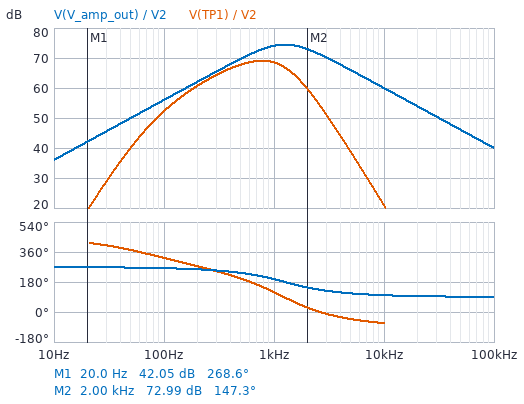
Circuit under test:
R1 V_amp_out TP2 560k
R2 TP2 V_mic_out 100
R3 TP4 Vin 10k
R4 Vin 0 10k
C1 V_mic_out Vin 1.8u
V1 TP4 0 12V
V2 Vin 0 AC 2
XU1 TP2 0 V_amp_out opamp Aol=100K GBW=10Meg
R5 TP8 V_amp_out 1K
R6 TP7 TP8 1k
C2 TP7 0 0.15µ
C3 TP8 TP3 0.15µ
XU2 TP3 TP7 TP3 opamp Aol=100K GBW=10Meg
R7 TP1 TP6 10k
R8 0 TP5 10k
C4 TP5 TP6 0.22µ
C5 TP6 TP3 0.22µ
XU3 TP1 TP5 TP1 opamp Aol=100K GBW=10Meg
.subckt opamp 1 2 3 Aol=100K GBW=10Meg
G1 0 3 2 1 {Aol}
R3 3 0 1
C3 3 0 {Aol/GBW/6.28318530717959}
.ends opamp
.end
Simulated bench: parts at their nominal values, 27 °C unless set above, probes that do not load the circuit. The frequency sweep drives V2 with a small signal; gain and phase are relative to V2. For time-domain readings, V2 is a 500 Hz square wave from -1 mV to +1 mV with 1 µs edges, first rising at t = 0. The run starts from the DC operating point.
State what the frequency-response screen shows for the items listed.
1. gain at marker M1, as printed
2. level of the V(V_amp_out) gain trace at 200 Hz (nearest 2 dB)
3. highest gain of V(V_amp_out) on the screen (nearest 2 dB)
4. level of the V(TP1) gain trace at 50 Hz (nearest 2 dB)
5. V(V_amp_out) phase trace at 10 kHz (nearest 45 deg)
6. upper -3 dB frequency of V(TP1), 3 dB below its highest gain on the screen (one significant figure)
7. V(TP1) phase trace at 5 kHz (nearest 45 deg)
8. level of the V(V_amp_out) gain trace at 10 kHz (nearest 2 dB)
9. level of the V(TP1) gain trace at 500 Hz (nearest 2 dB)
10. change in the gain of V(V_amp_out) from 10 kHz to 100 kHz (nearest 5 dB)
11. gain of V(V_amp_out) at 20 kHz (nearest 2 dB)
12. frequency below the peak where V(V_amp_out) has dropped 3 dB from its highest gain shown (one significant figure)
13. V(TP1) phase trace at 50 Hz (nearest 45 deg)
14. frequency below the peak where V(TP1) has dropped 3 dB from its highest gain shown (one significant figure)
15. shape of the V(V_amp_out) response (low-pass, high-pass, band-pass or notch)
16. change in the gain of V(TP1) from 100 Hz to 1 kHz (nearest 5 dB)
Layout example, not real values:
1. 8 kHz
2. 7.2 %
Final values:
1. 42.05 dB
2. 62 dB
3. 74 dB
4. 40 dB
5. 90 deg
6. 1 kHz
7. -45 deg
8. 60 dB
9. 68 dB
10. -20 dB
11. 54 dB
12. 600 Hz
13. 360 deg
14. 400 Hz
15. band-pass
16. 15 dB
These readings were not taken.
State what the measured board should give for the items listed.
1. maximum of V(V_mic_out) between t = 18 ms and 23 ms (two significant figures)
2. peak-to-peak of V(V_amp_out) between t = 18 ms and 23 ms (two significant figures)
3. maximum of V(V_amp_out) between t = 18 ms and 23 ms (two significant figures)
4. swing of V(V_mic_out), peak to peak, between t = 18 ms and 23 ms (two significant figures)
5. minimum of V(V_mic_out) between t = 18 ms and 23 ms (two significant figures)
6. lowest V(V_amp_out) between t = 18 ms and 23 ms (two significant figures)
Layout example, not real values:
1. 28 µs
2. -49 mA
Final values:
1. 2.0 mV
2. 14 V
3. 7.0 V
4. 4.0 mV
5. -2.0 mV
6. -7.0 V
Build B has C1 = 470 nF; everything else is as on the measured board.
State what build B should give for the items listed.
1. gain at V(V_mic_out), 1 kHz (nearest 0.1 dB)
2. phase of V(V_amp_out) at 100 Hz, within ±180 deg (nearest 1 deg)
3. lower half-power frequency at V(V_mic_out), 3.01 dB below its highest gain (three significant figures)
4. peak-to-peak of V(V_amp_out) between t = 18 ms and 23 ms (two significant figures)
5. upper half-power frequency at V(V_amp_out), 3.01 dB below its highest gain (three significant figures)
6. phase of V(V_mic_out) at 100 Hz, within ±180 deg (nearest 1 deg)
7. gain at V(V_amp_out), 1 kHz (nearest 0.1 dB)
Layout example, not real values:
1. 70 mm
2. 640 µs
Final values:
1. -8.0 dB
2. -92 deg
3. 1.92 kHz
4. 10 V
5. 3.58 kHz
6. 91 deg
7. 65.4 dB
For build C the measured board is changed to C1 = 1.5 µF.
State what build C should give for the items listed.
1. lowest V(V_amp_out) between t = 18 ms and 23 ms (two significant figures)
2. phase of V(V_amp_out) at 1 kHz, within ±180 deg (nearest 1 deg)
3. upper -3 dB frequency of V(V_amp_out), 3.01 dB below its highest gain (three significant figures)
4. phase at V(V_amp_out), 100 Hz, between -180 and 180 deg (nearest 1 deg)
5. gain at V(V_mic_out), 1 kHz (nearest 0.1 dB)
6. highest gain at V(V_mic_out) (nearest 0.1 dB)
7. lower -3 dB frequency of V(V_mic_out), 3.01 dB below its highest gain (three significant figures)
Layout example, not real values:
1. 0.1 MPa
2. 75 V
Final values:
1. -6.7 V
2. -155 deg
3. 2.61 kHz
4. -96 deg
5. 0.2 dB
6. 2.2 dB
7. 875 Hz
